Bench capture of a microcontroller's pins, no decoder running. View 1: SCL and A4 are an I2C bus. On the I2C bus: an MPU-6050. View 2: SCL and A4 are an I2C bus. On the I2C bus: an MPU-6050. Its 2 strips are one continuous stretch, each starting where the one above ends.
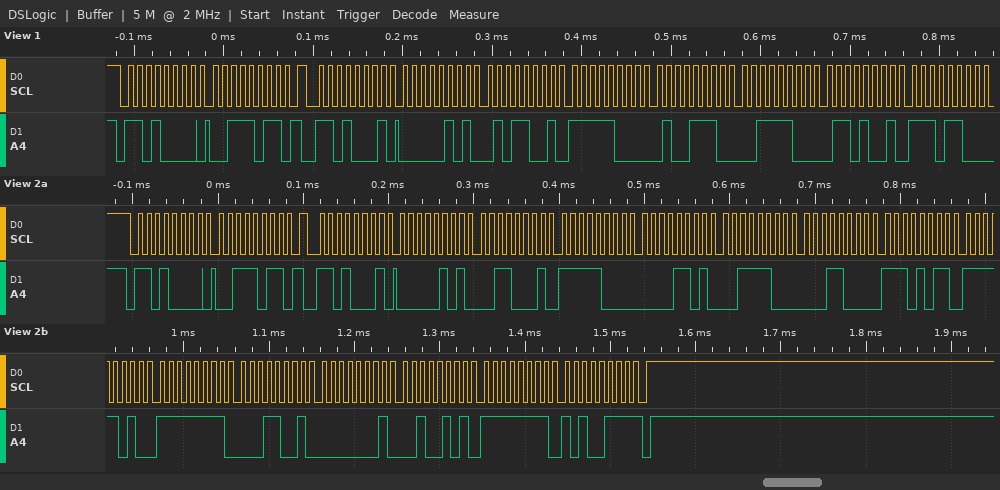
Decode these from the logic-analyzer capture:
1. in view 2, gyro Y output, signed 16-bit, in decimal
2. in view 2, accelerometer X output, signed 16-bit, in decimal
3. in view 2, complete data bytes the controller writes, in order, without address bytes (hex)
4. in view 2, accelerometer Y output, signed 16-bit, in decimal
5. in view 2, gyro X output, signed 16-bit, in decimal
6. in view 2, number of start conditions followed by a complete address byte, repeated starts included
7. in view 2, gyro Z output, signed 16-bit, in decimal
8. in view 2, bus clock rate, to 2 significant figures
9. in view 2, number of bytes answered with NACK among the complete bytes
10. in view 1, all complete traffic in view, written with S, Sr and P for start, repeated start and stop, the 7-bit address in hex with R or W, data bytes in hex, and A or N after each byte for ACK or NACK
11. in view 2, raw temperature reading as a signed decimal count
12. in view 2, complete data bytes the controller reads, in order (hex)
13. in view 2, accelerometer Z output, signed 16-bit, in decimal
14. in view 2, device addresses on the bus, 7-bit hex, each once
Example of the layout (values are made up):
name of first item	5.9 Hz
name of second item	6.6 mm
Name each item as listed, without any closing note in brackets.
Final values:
in view 2, gyro Y output, signed 16-bit, in decimal	293
in view 2, accelerometer X output, signed 16-bit, in decimal	1329
in view 2, complete data bytes the controller writes, in order, without address bytes	3B
in view 2, accelerometer Y output, signed 16-bit, in decimal	-2035
in view 2, gyro X output, signed 16-bit, in decimal	-231
in view 2, number of start conditions followed by a complete address byte, repeated starts included	2
in view 2, gyro Z output, signed 16-bit, in decimal	-89
in view 2, bus clock rate, to 2 significant figures	100 kHz
in view 2, number of bytes answered with NACK among the complete bytes	1
in view 1, all complete traffic in view, written with S, Sr and P for start, repeated start and stop, the 7-bit address in hex with R or W, data bytes in hex, and A or N after each byte for ACK or NACK	S 68W A 3B A Sr 68R A 05 A 59 A F8 A 4E A 3C A 69 A EC A
in view 2, raw temperature reading as a signed decimal count	-5126
in view 2, complete data bytes the controller reads, in order	05 31 F8 0D 3C 18 EB FA FF 19 01 25 FF A7
in view 2, accelerometer Z output, signed 16-bit, in decimal	15384
in view 2, device addresses on the bus, 7-bit hex, each once	0x68
